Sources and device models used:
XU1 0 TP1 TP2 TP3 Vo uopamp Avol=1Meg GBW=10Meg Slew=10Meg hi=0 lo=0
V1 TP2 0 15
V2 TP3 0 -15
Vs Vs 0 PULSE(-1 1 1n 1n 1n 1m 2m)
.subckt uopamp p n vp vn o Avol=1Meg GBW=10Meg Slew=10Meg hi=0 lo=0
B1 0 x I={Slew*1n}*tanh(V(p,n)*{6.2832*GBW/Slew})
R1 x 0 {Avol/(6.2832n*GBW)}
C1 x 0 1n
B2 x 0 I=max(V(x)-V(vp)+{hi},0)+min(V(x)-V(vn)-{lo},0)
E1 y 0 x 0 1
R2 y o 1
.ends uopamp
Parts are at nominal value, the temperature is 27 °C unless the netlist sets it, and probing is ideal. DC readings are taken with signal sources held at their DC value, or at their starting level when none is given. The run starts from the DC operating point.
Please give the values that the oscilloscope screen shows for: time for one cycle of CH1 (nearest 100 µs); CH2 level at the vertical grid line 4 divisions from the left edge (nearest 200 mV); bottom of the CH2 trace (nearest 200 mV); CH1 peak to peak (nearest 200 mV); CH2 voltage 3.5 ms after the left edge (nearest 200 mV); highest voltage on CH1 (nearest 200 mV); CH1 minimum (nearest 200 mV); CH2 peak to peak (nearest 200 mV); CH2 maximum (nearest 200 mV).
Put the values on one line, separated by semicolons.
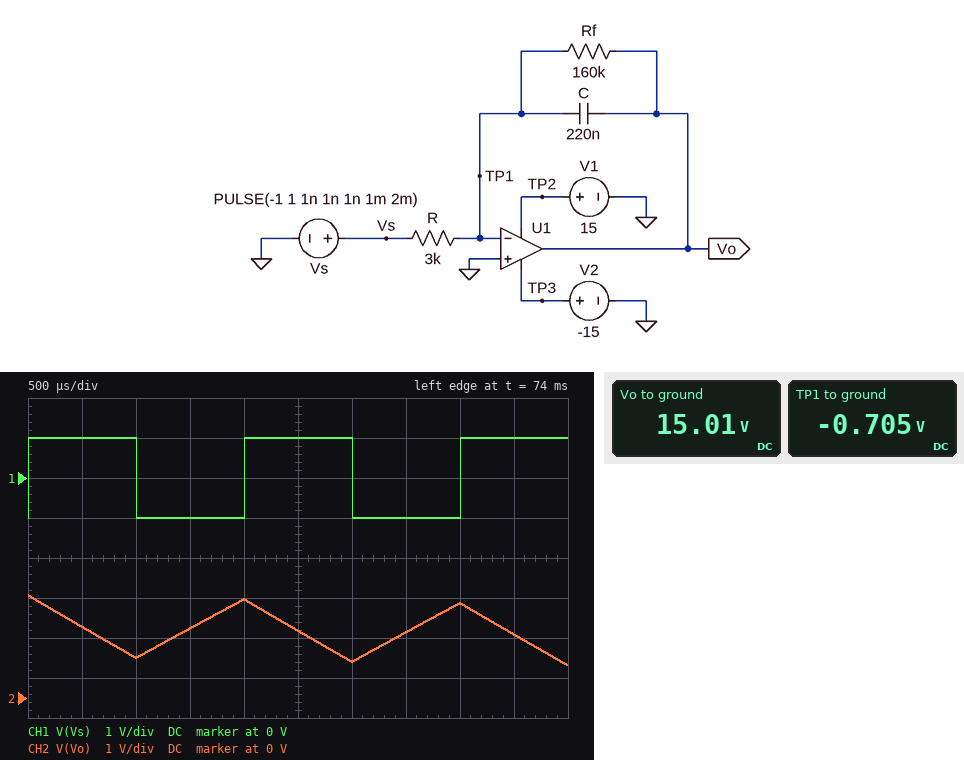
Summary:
2.0 ms; 2.4 V; 800 mV; 2.0 V; 1.6 V; 1.0 V; -1.0 V; 1.8 V; 2.6 V
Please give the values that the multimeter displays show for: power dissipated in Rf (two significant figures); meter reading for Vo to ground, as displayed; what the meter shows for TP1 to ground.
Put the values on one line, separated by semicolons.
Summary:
1.5 mW; 15.01 V; -0.705 V
